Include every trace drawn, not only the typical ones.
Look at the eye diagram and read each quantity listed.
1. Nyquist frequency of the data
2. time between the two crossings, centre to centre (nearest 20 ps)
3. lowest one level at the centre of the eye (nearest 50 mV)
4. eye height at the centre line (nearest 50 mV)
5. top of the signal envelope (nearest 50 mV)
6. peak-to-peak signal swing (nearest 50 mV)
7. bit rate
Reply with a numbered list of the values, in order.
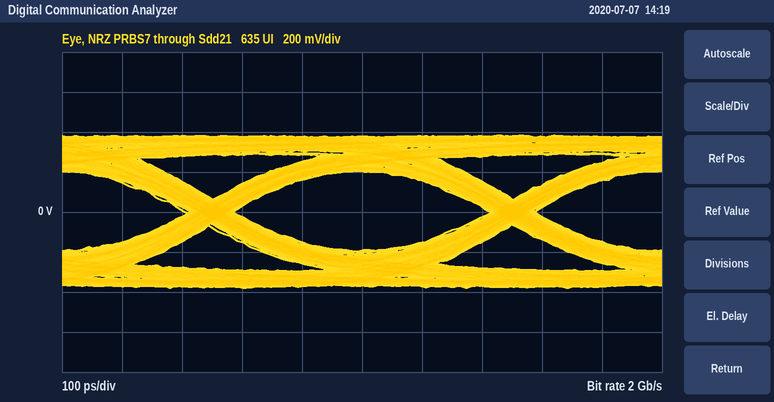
1. 1 GHz
2. 500 ps
3. 200 mV
4. 400 mV
5. 400 mV
6. 750 mV
7. 2 Gb/s
